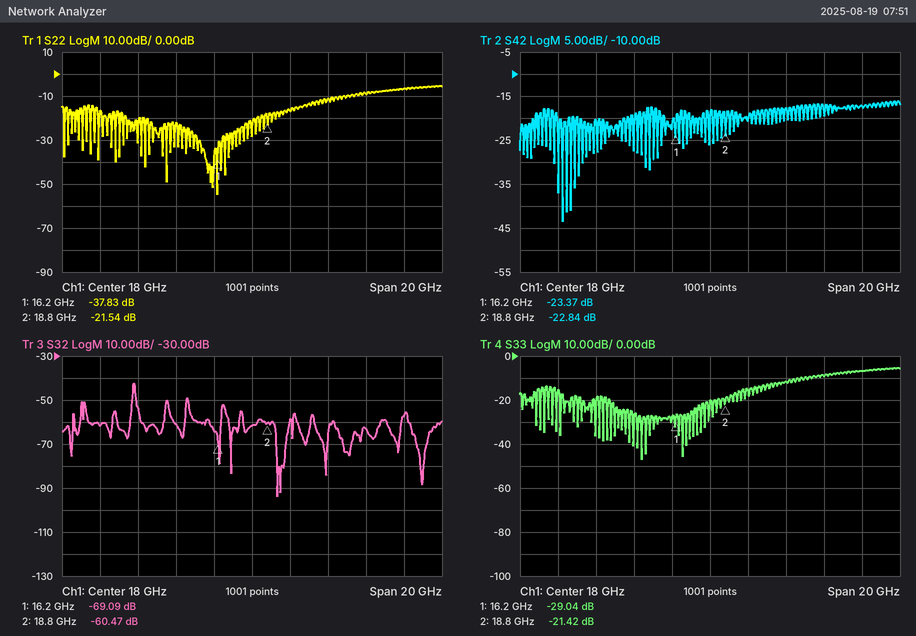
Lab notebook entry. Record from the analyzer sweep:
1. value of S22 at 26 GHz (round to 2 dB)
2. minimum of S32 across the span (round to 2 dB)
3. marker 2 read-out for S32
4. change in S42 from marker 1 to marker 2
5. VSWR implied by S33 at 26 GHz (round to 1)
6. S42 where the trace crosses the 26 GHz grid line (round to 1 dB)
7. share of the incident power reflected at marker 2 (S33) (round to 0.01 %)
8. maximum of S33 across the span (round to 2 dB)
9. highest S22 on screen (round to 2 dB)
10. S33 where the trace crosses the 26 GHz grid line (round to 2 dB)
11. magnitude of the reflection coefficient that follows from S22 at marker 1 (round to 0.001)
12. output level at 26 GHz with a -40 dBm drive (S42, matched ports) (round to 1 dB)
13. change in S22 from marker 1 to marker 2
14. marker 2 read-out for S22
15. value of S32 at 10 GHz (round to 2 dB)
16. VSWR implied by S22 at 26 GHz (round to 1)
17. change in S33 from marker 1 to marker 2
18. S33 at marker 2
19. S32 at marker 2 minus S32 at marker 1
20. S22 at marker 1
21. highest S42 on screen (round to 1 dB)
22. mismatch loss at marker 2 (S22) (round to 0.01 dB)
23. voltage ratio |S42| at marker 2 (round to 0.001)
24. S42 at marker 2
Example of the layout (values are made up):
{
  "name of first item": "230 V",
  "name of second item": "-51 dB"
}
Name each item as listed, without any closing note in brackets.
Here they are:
{
  "value of S22 at 26 GHz": "-6 dB",
  "minimum of S32 across the span": "-94 dB",
  "marker 2 read-out for S32": "-60.47 dB",
  "change in S42 from marker 1 to marker 2": "0.53 dB",
  "VSWR implied by S33 at 26 GHz": "3",
  "S42 where the trace crosses the 26 GHz grid line": "-17 dB",
  "share of the incident power reflected at marker 2 (S33)": "0.72 %",
  "maximum of S33 across the span": "-6 dB",
  "highest S22 on screen": "-6 dB",
  "S33 where the trace crosses the 26 GHz grid line": "-6 dB",
  "magnitude of the reflection coefficient that follows from S22 at marker 1": "0.013",
  "output level at 26 GHz with a -40 dBm drive (S42, matched ports)": "-57 dBm",
  "change in S22 from marker 1 to marker 2": "16.29 dB",
  "marker 2 read-out for S22": "-21.54 dB",
  "value of S32 at 10 GHz": "-62 dB",
  "VSWR implied by S22 at 26 GHz": "3",
  "change in S33 from marker 1 to marker 2": "7.62 dB",
  "S33 at marker 2": "-21.42 dB",
  "S32 at marker 2 minus S32 at marker 1": "8.62 dB",
  "S22 at marker 1": "-37.83 dB",
  "highest S42 on screen": "-16 dB",
  "mismatch loss at marker 2 (S22)": "0.03 dB",
  "voltage ratio |S42| at marker 2": "0.072",
  "S42 at marker 2": "-22.84 dB"
}
